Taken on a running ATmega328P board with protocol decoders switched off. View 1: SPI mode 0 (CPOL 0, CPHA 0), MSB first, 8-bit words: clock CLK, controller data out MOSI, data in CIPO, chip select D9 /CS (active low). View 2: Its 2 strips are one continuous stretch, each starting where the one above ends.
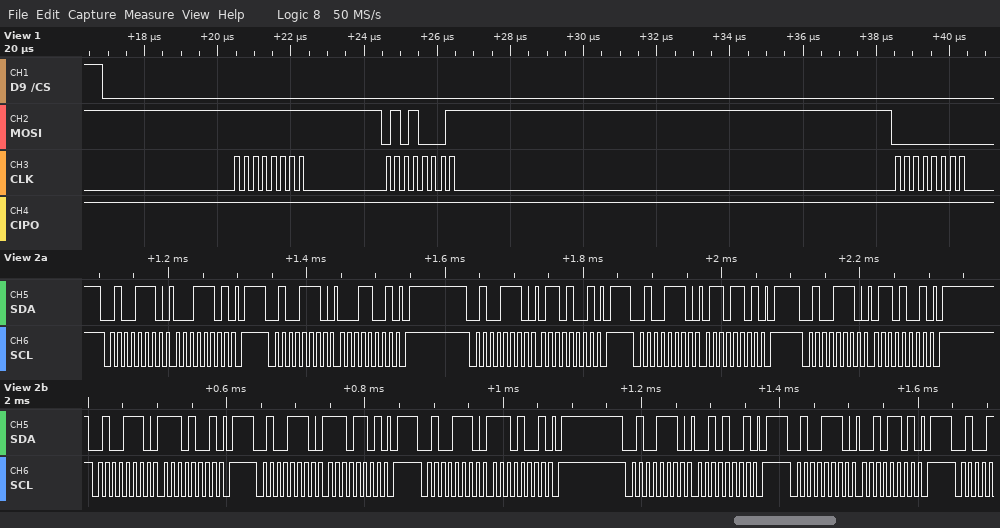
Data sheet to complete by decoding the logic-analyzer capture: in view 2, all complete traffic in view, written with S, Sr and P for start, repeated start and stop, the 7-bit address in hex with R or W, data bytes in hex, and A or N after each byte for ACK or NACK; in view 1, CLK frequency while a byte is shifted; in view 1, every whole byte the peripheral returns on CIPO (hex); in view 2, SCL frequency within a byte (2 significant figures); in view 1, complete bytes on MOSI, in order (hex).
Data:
S 27W A 1D A P S 27W A 19 A P S 27W A 69 A P S 27W A 6D A P S 27W A 69 A P S 27W A E9 A P S 27W A ED A P S 27W A E9 A P S 27W A 29 A P S 27W A 2D A P
4 MHz
FF FF FF
100 kHz
FF 51 00
